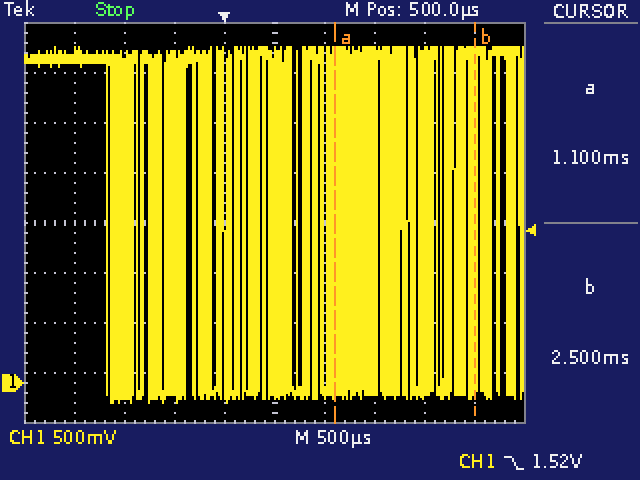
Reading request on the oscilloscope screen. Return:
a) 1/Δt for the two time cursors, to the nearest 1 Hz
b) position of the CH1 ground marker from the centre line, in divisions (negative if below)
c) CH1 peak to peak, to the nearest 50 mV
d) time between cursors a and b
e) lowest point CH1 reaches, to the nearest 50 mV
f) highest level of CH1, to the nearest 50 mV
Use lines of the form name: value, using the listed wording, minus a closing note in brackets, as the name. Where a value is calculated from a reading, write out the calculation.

1/Δt for the two time cursors, to the nearest 1 Hz: 1 / 1.40 ms ≈ 714 Hz
position of the CH1 ground marker from the centre line, in divisions: -3.2 div
CH1 peak to peak, to the nearest 50 mV: 3.35 V − (-200 mV) = 3.55 V
time between cursors a and b: 2.5 ms − (1.1 ms) = 1.40 ms
lowest point CH1 reaches, to the nearest 50 mV: -200 mV
highest level of CH1, to the nearest 50 mV: 3.35 V
